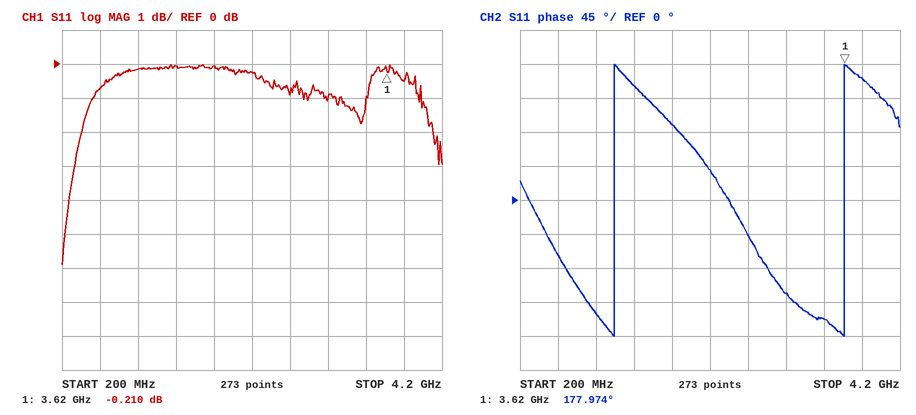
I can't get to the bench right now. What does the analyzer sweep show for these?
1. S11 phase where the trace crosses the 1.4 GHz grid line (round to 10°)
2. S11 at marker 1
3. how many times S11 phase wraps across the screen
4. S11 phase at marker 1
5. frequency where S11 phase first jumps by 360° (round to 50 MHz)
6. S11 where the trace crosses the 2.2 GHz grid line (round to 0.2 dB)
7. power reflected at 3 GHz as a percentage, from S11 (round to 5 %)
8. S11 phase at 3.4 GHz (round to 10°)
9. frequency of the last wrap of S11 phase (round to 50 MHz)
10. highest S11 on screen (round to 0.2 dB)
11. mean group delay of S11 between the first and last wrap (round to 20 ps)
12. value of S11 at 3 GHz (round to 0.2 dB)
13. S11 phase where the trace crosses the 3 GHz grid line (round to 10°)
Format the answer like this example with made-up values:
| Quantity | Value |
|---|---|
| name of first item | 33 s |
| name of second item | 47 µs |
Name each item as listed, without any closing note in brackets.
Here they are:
| Quantity | Value |
|---|---|
| S11 phase where the trace crosses the 1.4 GHz grid line | 150° |
| S11 at marker 1 | -0.210 dB |
| how many times S11 phase wraps across the screen | 2 |
| S11 phase at marker 1 | 177.974° |
| frequency where S11 phase first jumps by 360° | 1.20 GHz |
| S11 where the trace crosses the 2.2 GHz grid line | -0.2 dB |
| power reflected at 3 GHz as a percentage, from S11 | 80 % |
| S11 phase at 3.4 GHz | -160° |
| frequency of the last wrap of S11 phase | 3.60 GHz |
| highest S11 on screen | 0.0 dB |
| mean group delay of S11 between the first and last wrap | 420 ps |
| value of S11 at 3 GHz | -1.0 dB |
| S11 phase where the trace crosses the 3 GHz grid line | -120° |
